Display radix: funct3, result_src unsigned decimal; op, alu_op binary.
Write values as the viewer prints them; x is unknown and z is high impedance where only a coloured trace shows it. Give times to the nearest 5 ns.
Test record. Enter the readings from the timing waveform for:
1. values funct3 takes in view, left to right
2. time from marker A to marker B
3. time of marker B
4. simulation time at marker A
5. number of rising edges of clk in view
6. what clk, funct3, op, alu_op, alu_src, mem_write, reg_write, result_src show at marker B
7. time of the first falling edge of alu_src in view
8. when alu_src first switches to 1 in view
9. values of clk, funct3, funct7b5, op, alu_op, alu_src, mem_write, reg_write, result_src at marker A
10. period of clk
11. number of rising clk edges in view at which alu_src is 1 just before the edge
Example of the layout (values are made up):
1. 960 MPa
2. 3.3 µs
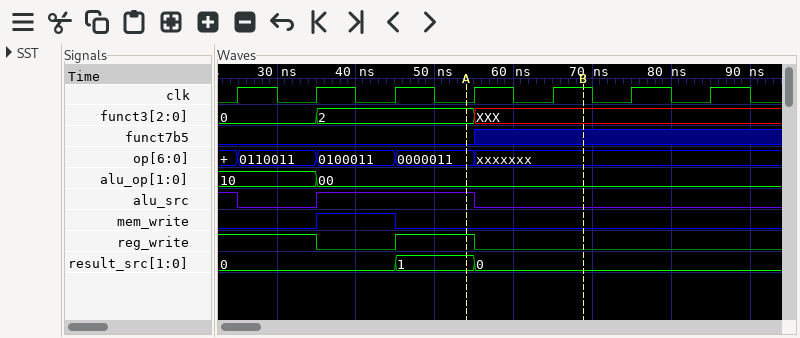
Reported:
1. 0, 2, XXX
2. 15 ns
3. 70 ns
4. 55 ns
5. 7
6. clk=1, funct3=XXX, op=xxxxxxx, alu_op=00, alu_src=0, mem_write=0, reg_write=0, result_src=0
7. 25 ns
8. 35 ns
9. clk=0, funct3=2, funct7b5=0, op=0000011, alu_op=00, alu_src=1, mem_write=0, reg_write=1, result_src=1
10. 10 ns
11. 3
